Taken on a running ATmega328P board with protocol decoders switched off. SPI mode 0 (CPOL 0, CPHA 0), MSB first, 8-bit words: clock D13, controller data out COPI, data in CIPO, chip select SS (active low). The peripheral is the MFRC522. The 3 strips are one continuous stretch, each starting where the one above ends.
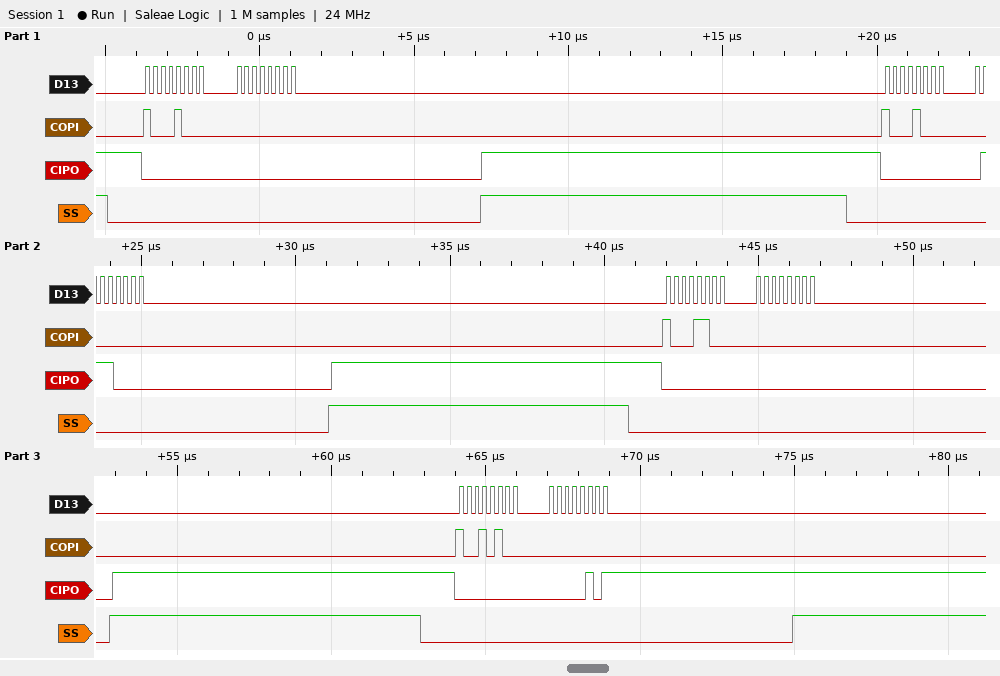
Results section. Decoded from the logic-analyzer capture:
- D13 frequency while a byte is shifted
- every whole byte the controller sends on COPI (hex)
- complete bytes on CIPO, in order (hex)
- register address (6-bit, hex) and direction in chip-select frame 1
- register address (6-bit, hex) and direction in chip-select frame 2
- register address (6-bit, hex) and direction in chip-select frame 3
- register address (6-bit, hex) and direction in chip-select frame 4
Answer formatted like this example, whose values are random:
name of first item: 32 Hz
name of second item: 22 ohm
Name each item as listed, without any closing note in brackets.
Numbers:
D13 frequency while a byte is shifted: 4 MHz
every whole byte the controller sends on COPI: 88 00 88 00 8C 00 94 00
complete bytes on CIPO, in order: 00 00 00 70 00 00 00 05
register address (6-bit, hex) and direction in chip-select frame 1: 0x04 read
register address (6-bit, hex) and direction in chip-select frame 2: 0x04 read
register address (6-bit, hex) and direction in chip-select frame 3: 0x06 read
register address (6-bit, hex) and direction in chip-select frame 4: 0x0A read
